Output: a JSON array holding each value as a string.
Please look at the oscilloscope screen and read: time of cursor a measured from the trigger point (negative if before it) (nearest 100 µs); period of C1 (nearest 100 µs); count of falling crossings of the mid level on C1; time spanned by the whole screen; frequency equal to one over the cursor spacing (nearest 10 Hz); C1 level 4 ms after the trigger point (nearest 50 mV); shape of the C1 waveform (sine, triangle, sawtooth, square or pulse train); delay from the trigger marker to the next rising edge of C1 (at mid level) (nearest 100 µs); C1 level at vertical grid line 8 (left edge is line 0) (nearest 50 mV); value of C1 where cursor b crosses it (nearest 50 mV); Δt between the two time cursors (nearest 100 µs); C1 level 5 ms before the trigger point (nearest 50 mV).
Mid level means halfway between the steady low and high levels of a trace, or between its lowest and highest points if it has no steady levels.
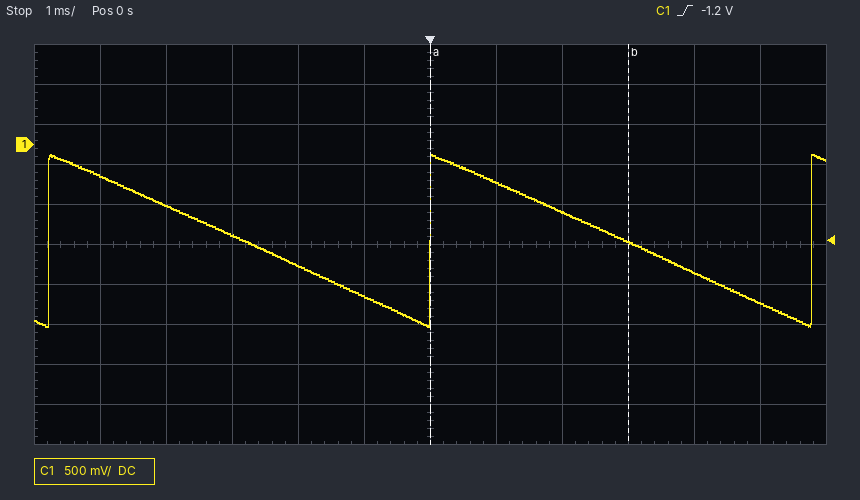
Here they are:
["0.0 ms", "5.8 ms", "2", "12 ms", "330 Hz", "-1.60 V", "sawtooth", "5.8 ms", "-850 mV", "-1.20 V", "3.0 ms", "-400 mV"]
